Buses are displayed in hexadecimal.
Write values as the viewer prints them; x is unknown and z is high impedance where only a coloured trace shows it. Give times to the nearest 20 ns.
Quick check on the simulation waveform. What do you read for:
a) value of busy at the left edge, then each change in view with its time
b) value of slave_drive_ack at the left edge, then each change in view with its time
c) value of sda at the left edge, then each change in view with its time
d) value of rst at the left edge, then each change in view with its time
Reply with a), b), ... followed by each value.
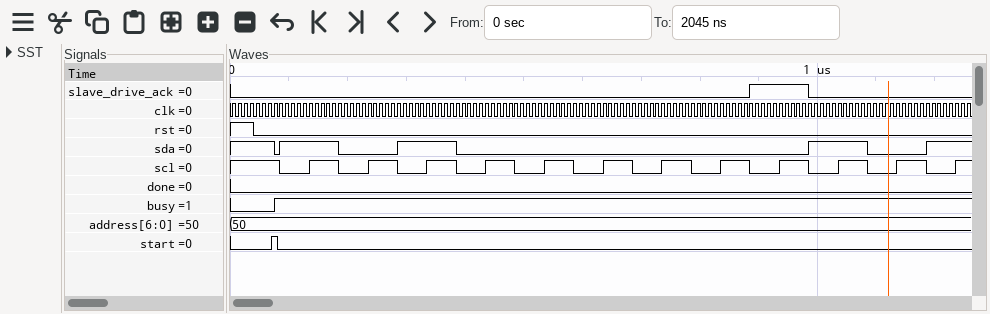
a) 0, 1 at 80 ns
b) 0, 1 at 880 ns, 0 at 980 ns
c) 1, 0 at 80 ns, 1 at 80 ns, 0 at 180 ns, 1 at 280 ns, 0 at 380 ns, 1 at 980 ns, 0 at 1080 ns, 1 at 1180 ns
d) 1, 0 at 40 ns
